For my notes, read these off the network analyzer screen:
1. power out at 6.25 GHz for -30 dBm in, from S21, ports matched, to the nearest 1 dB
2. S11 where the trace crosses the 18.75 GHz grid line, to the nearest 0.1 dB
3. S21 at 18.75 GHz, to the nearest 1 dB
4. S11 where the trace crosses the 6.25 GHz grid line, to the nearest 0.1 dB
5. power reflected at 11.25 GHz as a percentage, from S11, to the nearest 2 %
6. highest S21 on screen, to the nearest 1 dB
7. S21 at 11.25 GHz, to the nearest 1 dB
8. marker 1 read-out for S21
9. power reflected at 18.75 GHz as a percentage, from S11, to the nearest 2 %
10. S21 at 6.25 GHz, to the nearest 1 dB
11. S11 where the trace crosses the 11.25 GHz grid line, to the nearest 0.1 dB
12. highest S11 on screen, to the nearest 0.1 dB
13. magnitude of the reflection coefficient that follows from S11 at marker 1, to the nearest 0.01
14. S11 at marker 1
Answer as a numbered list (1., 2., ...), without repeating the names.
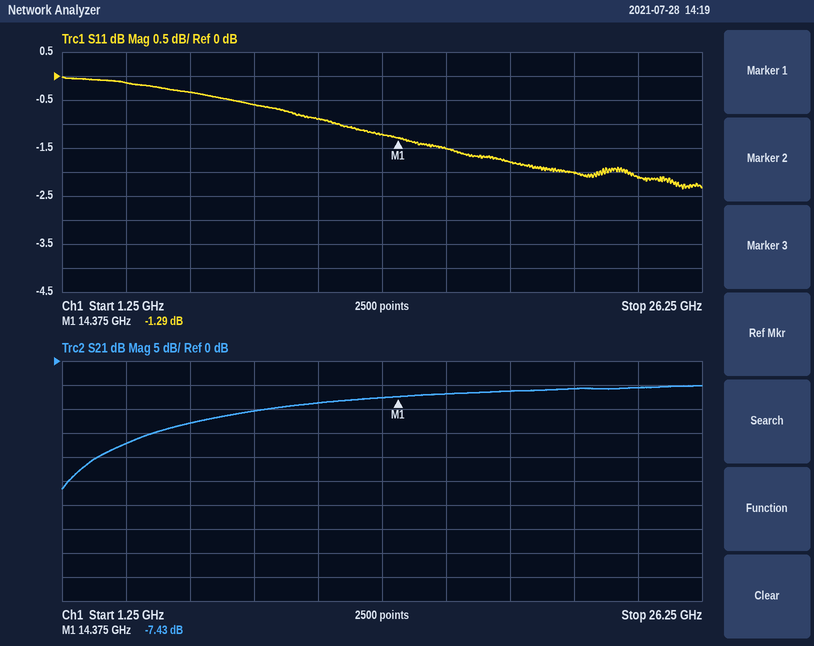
1. -43 dBm
2. -1.8 dB
3. -6 dB
4. -0.3 dB
5. 82 %
6. -5 dB
7. -9 dB
8. -7.43 dB
9. 66 %
10. -13 dB
11. -0.9 dB
12. 0.0 dB
13. 0.86
14. -1.29 dB
